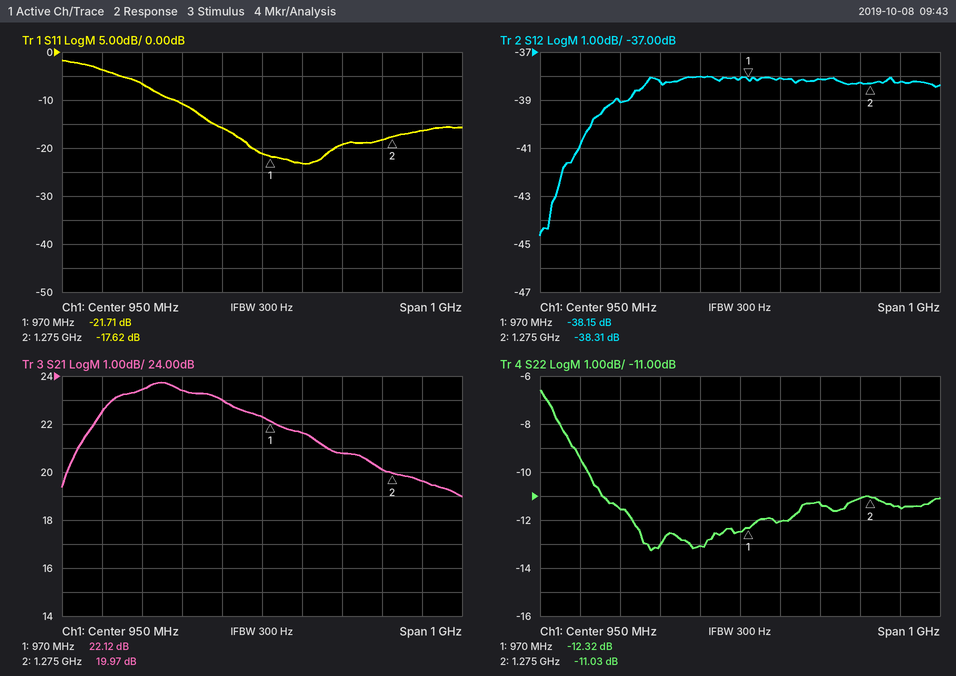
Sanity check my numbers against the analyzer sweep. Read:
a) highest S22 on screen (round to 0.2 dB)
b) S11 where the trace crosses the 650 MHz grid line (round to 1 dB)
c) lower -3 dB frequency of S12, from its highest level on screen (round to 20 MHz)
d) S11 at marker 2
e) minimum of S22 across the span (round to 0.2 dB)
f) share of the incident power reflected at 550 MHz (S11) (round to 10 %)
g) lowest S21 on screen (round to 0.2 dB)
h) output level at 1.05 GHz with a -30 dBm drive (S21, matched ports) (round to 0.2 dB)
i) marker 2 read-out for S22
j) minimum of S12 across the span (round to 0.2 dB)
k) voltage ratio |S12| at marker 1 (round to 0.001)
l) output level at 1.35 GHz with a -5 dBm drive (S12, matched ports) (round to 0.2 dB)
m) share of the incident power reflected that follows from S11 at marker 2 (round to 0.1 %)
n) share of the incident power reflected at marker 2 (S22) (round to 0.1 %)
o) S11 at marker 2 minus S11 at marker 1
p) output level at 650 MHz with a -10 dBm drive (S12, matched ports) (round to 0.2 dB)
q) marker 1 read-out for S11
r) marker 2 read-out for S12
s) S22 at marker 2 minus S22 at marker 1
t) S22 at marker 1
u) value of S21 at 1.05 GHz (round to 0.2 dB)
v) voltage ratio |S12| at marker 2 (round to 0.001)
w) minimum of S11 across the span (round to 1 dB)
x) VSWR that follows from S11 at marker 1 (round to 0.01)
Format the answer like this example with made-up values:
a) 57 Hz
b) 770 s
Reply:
a) -6.6 dB
b) -7 dB
c) 540 MHz
d) -17.62 dB
e) -13.2 dB
f) 40 %
g) 19.0 dB
h) -8.4 dBm
i) -11.03 dB
j) -44.6 dB
k) 0.012
l) -43.2 dBm
m) 1.7 %
n) 7.9 %
o) 4.09 dB
p) -49.0 dBm
q) -21.71 dB
r) -38.31 dB
s) 1.29 dB
t) -12.32 dB
u) 21.6 dB
v) 0.012
w) -23 dB
x) 1.18
